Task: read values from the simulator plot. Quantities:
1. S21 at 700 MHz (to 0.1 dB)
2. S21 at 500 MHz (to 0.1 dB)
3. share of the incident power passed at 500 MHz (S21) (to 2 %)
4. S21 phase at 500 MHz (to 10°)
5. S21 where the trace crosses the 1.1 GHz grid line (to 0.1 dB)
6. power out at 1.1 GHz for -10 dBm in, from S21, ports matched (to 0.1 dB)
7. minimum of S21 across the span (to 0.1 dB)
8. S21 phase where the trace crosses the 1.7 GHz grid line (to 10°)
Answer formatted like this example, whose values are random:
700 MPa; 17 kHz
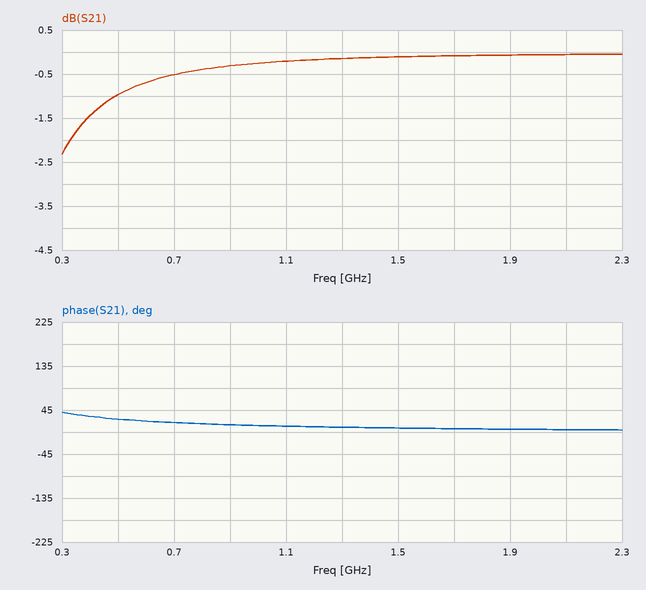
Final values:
-0.5 dB; -1.0 dB; 80 %; 30°; -0.2 dB; -10.2 dBm; -2.3 dB; 10°
